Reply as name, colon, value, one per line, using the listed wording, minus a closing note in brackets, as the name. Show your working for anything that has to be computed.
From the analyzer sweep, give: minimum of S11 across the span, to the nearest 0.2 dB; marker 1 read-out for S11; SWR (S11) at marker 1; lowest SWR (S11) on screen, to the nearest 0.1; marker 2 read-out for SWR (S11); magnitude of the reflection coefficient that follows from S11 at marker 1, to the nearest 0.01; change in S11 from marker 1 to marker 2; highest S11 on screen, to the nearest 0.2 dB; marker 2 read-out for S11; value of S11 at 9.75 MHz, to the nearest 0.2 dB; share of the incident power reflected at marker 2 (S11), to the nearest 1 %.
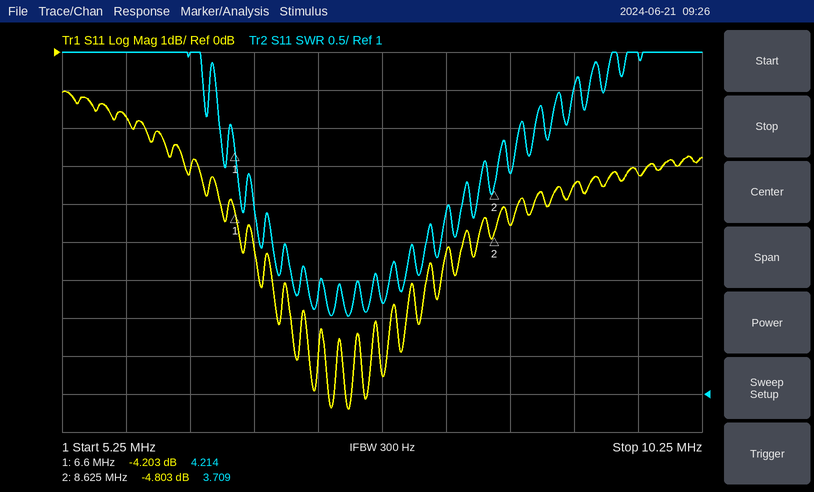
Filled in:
minimum of S11 across the span, to the nearest 0.2 dB: -9.4 dB
marker 1 read-out for S11: -4.203 dB
SWR (S11) at marker 1: 4.214
lowest SWR (S11) on screen, to the nearest 0.1: 2.0
marker 2 read-out for SWR: 3.709
magnitude of the reflection coefficient that follows from S11 at marker 1, to the nearest 0.01: 10^(-4.203/20) ≈ 0.62
change in S11 from marker 1 to marker 2: -4.803 − (-4.203) = -0.600 dB
highest S11 on screen, to the nearest 0.2 dB: -1.0 dB
marker 2 read-out for S11: -4.803 dB
value of S11 at 9.75 MHz, to the nearest 0.2 dB: -3.2 dB
share of the incident power reflected at marker 2 (S11), to the nearest 1 %: 10^(-4.803/10) ≈ 33 %
